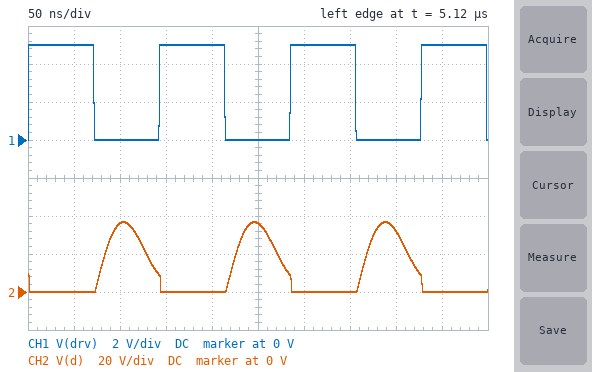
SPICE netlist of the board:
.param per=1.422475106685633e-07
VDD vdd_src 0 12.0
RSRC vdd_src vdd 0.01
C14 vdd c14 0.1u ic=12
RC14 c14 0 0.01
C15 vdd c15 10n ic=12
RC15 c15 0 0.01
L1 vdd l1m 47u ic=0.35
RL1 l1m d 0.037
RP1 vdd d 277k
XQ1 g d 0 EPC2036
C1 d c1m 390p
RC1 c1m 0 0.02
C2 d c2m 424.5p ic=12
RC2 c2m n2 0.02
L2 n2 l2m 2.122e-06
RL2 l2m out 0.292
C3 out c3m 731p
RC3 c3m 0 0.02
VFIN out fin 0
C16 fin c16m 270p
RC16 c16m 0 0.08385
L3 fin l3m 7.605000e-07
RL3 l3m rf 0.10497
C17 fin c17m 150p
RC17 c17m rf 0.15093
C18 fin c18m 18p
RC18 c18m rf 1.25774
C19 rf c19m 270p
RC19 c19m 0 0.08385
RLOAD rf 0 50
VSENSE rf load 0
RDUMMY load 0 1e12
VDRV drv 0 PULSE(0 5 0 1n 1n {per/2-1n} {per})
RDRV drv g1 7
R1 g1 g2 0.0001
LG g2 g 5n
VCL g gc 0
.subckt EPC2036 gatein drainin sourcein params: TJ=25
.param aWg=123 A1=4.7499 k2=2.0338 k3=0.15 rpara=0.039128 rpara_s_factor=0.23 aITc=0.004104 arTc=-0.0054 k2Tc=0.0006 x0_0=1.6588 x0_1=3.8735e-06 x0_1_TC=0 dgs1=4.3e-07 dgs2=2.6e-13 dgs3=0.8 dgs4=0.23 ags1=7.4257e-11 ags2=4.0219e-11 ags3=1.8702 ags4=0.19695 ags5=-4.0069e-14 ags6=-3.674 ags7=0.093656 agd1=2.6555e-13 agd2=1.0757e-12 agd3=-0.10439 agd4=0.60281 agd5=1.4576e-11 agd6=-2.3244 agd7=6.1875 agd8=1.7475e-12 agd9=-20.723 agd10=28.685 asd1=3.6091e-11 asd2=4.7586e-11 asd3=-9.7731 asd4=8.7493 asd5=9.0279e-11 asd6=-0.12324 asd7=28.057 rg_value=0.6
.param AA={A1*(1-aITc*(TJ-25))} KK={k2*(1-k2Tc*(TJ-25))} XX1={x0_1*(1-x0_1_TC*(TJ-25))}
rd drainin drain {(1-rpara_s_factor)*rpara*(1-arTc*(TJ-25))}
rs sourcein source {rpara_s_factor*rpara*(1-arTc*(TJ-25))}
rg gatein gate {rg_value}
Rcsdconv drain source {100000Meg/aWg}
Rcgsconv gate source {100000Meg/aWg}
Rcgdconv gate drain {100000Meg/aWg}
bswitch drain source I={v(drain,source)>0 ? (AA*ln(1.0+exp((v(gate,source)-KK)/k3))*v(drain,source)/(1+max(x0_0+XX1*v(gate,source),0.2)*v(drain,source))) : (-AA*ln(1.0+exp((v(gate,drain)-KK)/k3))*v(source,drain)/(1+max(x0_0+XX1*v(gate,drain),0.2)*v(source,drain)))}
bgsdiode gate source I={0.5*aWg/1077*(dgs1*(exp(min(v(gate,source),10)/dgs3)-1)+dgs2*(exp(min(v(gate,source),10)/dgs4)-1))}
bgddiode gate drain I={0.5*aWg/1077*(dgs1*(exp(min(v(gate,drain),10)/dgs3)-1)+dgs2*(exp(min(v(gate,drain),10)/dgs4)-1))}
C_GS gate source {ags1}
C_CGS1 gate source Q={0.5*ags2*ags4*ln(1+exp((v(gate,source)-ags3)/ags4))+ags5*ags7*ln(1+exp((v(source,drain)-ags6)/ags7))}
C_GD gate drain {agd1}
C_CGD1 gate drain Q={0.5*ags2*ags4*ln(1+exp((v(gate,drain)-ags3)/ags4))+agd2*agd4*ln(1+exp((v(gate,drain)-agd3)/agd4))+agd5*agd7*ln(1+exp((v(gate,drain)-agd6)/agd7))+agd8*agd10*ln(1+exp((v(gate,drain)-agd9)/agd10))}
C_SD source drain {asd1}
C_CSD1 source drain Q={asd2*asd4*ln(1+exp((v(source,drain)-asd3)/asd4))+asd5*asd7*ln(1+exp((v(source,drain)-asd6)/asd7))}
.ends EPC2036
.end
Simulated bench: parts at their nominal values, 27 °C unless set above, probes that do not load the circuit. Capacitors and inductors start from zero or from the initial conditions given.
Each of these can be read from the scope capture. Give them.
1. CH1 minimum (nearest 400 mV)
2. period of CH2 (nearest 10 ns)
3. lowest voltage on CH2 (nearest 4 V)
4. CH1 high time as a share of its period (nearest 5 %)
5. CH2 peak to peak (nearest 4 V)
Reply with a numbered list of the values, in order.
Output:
1. 0 V
2. 140 ns
3. 0 V
4. 50 %
5. 36 V
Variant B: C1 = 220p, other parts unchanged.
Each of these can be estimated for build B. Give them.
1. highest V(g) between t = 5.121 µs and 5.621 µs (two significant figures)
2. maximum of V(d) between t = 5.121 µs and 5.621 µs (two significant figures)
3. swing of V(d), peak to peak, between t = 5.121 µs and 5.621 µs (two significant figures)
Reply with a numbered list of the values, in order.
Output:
1. 5.5 V
2. 46 V
3. 47 V
